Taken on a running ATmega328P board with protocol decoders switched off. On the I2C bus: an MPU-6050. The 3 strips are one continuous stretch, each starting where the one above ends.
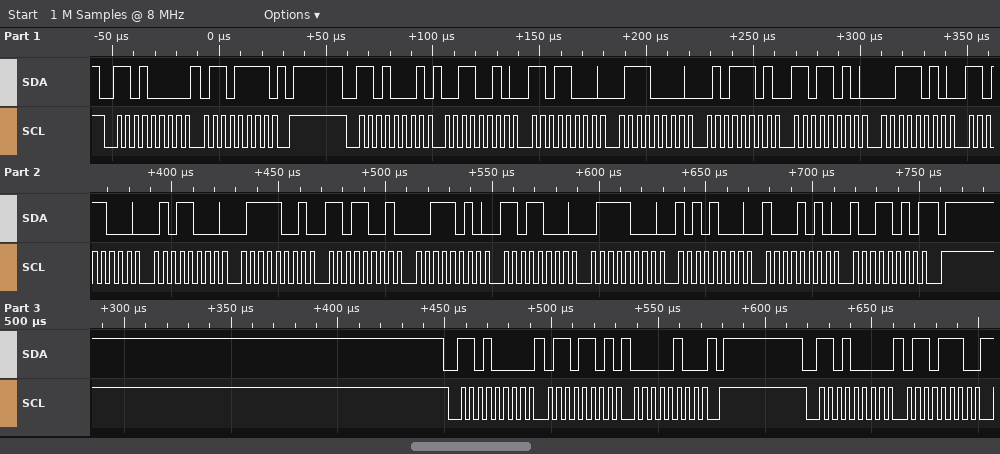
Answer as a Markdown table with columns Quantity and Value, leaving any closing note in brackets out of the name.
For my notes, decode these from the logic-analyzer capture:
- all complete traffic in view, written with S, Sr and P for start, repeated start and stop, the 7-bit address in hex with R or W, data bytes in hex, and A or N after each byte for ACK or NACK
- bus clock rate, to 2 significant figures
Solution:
| Quantity | Value |
|---|---|
| all complete traffic in view, written with S, Sr and P for start, repeated start and stop, the 7-bit address in hex with R or W, data bytes in hex, and A or N after each byte for ACK or NACK | S 68W A 6F A P S 68R A 32 A D8 A 70 A 5D A DA A 3A A D8 A 58 A 79 A D9 A 3A A D8 A 78 A A8 A 8A A 9A N P S 68W A 6D A 04 A P S 68W A 6E A |
| bus clock rate, to 2 significant figures | 250 kHz |
